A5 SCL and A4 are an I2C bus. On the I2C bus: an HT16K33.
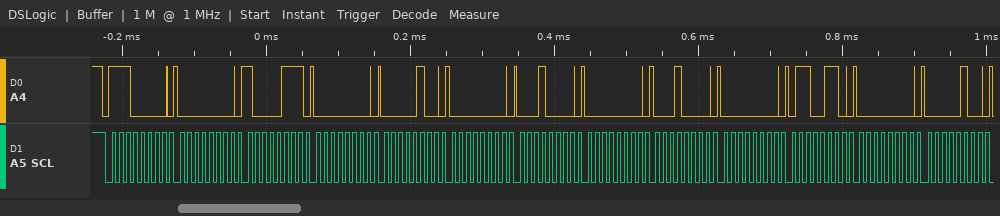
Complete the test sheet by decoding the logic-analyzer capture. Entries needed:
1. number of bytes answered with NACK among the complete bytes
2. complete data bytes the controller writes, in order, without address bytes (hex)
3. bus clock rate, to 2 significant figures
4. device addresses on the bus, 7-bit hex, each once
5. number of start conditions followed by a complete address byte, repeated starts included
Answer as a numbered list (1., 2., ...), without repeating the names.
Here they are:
1. 0
2. 00 87 00 04 00 10 00 10 00 66 00 04
3. 100 kHz
4. 0x70
5. 1
